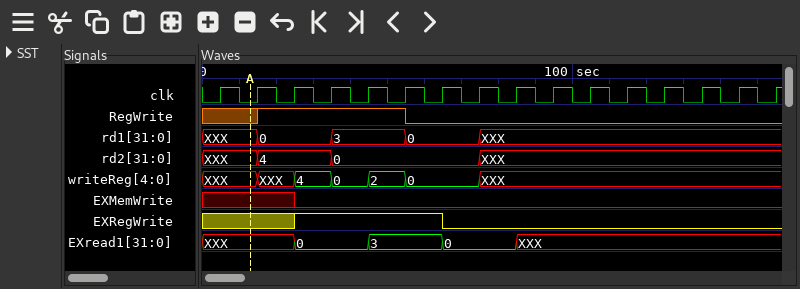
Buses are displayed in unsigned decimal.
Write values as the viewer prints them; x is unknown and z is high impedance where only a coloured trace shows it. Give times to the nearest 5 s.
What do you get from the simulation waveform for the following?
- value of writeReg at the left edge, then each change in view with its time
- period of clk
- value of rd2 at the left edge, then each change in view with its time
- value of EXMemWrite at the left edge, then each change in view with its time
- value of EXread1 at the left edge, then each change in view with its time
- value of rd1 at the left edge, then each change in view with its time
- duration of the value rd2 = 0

XXX, XXX at 15 s, 4 at 25 s, 0 at 35 s, 2 at 45 s, 0 at 55 s, XXX at 75 s
10 s
XXX, 4 at 15 s, 0 at 35 s, XXX at 75 s
x, 0 at 25 s
XXX, 0 at 25 s, 3 at 45 s, 0 at 65 s, XXX at 85 s
XXX, 0 at 15 s, 3 at 35 s, 0 at 55 s, XXX at 75 s
40 s
